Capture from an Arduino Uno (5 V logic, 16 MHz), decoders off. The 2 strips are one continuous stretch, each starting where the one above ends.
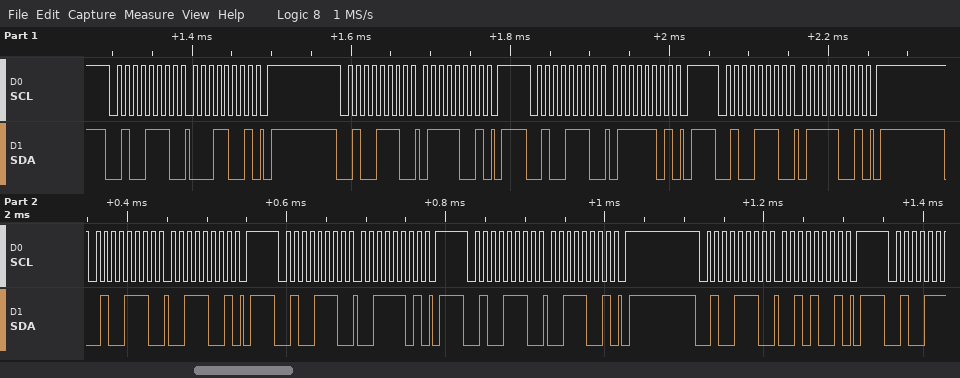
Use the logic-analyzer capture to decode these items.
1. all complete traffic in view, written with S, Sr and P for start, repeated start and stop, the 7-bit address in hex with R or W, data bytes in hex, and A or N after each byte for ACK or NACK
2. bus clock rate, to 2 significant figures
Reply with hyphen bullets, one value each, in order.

- S 27W A 19 A P S 27W A 79 A P S 27W A 7D A P S 27W A 79 A P S 27W A 39 A P S 27W A 3D A P S 27W A 39 A P S 27W A 29 A P
- 100 kHz
